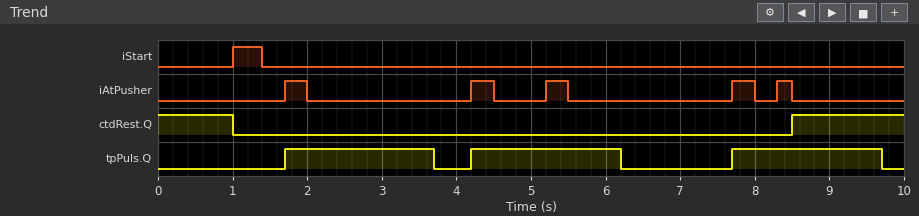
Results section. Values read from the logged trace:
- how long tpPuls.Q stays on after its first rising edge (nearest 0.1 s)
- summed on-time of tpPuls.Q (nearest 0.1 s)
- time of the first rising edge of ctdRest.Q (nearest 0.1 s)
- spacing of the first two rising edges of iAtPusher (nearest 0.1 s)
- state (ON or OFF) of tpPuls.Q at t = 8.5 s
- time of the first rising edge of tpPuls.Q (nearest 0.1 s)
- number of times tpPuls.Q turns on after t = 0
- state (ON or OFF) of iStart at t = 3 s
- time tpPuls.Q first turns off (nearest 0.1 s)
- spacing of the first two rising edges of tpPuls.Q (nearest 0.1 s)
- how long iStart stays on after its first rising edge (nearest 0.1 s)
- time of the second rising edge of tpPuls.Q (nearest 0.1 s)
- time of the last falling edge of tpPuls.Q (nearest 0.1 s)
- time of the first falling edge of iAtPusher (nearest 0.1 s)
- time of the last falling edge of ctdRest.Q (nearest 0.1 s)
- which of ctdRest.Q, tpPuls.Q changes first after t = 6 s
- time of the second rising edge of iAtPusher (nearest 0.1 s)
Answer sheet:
2.0 s
6.0 s
8.5 s
2.5 s
ON
1.7 s
3
OFF
3.7 s
2.5 s
0.4 s
4.2 s
9.7 s
2.0 s
1.0 s
tpPuls.Q
4.2 s
